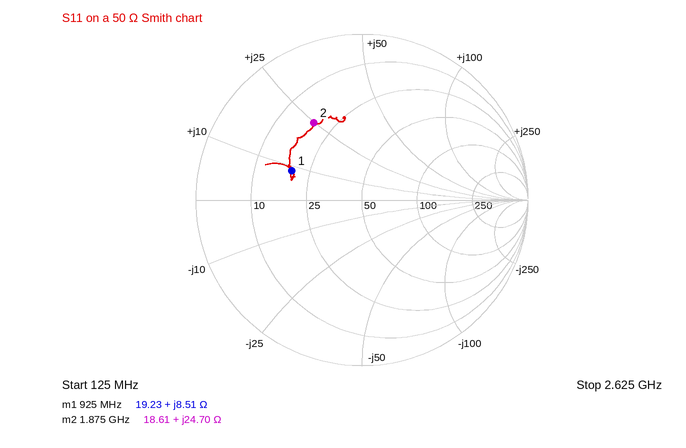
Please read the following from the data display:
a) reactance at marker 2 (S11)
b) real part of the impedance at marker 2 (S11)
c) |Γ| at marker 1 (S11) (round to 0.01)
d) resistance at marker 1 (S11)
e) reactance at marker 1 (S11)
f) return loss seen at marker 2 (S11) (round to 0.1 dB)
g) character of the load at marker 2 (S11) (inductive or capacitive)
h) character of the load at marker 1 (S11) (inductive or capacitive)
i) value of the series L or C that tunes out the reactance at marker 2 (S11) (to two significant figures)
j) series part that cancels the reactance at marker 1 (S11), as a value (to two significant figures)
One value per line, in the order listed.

+24.70 Ω
18.61 Ω
0.46
19.23 Ω
+8.51 Ω
5.2 dB
inductive
inductive
3.4 pF
20 pF
